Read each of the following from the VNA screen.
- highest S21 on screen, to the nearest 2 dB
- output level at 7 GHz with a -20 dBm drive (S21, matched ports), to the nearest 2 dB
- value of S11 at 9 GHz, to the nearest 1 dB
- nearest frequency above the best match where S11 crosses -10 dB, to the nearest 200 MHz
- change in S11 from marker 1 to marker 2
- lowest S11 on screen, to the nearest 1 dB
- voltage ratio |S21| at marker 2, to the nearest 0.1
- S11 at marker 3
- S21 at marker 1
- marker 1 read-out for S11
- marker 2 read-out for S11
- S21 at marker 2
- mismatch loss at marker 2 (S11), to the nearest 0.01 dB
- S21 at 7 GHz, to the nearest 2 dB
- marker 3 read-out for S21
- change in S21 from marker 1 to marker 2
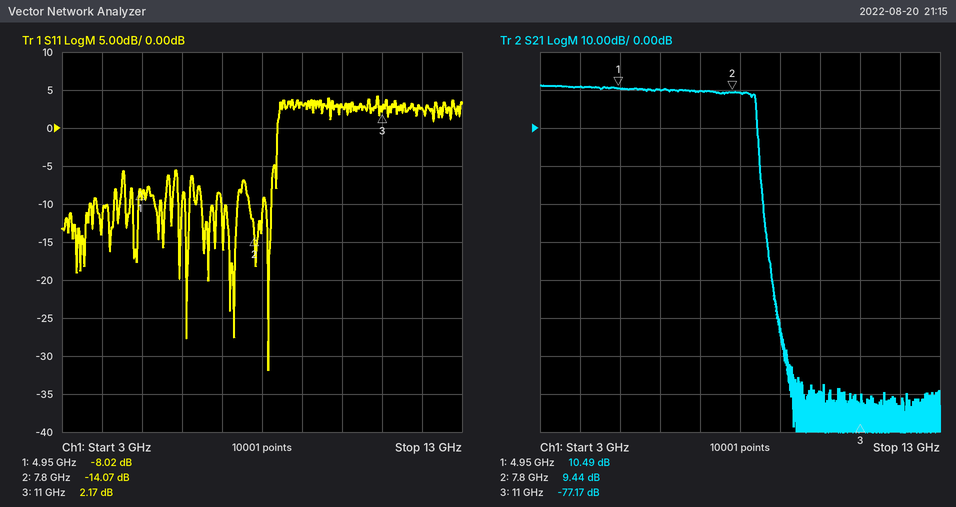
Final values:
12 dB
-10 dBm
3 dB
8.2 GHz
-6.05 dB
-32 dB
3.0
2.17 dB
10.49 dB
-8.02 dB
-14.07 dB
9.44 dB
0.17 dB
10 dB
-77.17 dB
-1.05 dB
